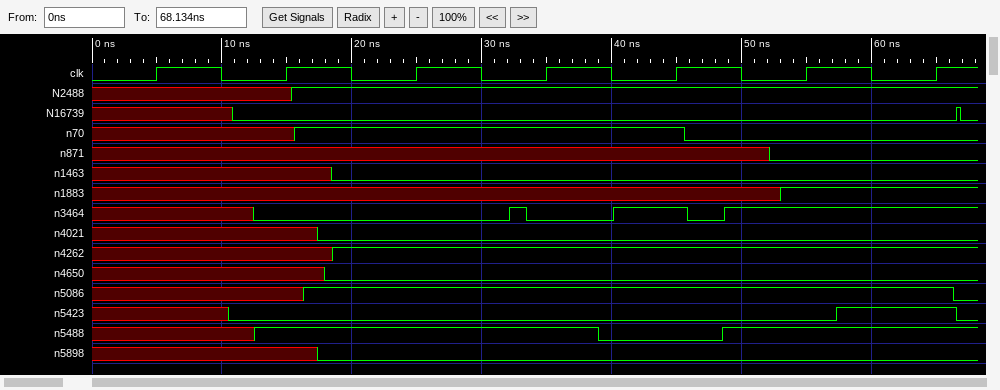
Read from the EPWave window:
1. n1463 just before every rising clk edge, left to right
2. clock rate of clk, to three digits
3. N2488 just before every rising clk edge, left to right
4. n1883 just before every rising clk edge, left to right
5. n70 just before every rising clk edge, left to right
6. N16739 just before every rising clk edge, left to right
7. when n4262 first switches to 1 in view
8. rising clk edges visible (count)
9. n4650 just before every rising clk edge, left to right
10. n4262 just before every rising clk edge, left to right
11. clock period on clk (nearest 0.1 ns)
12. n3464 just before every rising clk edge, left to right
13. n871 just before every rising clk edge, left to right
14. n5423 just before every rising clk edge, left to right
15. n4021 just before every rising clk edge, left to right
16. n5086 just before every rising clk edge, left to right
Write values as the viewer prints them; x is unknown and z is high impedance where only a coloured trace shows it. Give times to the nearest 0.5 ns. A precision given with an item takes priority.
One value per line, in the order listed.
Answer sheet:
x x 0 0 0 0 0
100 MHz
x x 1 1 1 1 1
x x x x x 1 1
x x 1 1 1 0 0
x 0 0 0 0 0 0
18.5 ns
7
x x 0 0 0 0 0
x x 1 1 1 1 1
10 ns
x 0 0 0 1 1 1
x x x x x 0 0
x 0 0 0 0 0 1
x x 0 0 0 0 0
x x 1 1 1 1 1
